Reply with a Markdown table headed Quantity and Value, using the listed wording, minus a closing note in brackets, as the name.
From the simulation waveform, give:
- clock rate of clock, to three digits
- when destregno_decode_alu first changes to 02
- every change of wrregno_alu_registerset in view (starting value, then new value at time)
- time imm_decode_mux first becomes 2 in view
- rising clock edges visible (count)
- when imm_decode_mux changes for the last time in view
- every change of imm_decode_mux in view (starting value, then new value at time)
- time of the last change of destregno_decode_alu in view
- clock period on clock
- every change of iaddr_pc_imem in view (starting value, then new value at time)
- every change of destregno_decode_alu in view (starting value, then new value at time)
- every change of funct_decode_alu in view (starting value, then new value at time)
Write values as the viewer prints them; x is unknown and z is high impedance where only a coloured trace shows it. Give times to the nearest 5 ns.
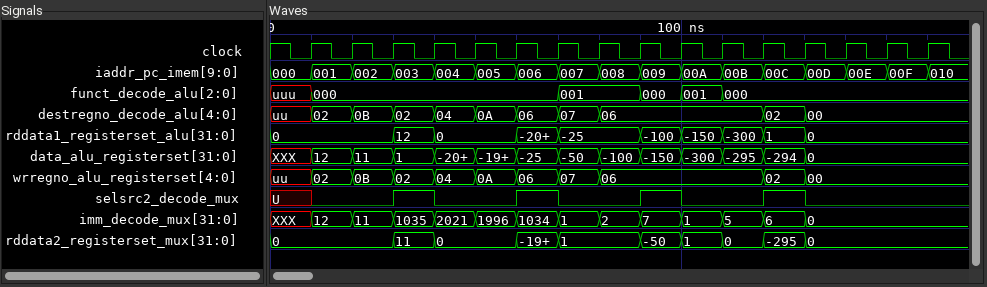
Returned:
| Quantity | Value |
|---|---|
| clock rate of clock, to three digits | 100 MHz |
| when destregno_decode_alu first changes to 02 | 10 ns |
| every change of wrregno_alu_registerset in view | uu, 02 at 10 ns, 0B at 20 ns, 02 at 30 ns, 04 at 40 ns, 0A at 50 ns, 06 at 60 ns, 07 at 70 ns, 06 at 80 ns, 02 at 120 ns, 00 at 130 ns |
| time imm_decode_mux first becomes 2 in view | 80 ns |
| rising clock edges visible | 16 |
| when imm_decode_mux changes for the last time in view | 130 ns |
| every change of imm_decode_mux in view | XXX, 12 at 10 ns, 11 at 20 ns, 1035 at 30 ns, 2021 at 40 ns, 1996 at 50 ns, 1034 at 60 ns, 1 at 70 ns, 2 at 80 ns, 7 at 90 ns, 1 at 100 ns, 5 at 110 ns, 6 at 120 ns, 0 at 130 ns |
| time of the last change of destregno_decode_alu in view | 130 ns |
| clock period on clock | 10 ns |
| every change of iaddr_pc_imem in view | 000, 001 at 10 ns, 002 at 20 ns, 003 at 30 ns, 004 at 40 ns, 005 at 50 ns, 006 at 60 ns, 007 at 70 ns, 008 at 80 ns, 009 at 90 ns, 00A at 100 ns, 00B at 110 ns, 00C at 120 ns, 00D at 130 ns, 00E at 140 ns, 00F at 150 ns, 010 at 160 ns |
| every change of destregno_decode_alu in view | uu, 02 at 10 ns, 0B at 20 ns, 02 at 30 ns, 04 at 40 ns, 0A at 50 ns, 06 at 60 ns, 07 at 70 ns, 06 at 80 ns, 02 at 120 ns, 00 at 130 ns |
| every change of funct_decode_alu in view | uuu, 000 at 10 ns, 001 at 70 ns, 000 at 90 ns, 001 at 100 ns, 000 at 110 ns |
